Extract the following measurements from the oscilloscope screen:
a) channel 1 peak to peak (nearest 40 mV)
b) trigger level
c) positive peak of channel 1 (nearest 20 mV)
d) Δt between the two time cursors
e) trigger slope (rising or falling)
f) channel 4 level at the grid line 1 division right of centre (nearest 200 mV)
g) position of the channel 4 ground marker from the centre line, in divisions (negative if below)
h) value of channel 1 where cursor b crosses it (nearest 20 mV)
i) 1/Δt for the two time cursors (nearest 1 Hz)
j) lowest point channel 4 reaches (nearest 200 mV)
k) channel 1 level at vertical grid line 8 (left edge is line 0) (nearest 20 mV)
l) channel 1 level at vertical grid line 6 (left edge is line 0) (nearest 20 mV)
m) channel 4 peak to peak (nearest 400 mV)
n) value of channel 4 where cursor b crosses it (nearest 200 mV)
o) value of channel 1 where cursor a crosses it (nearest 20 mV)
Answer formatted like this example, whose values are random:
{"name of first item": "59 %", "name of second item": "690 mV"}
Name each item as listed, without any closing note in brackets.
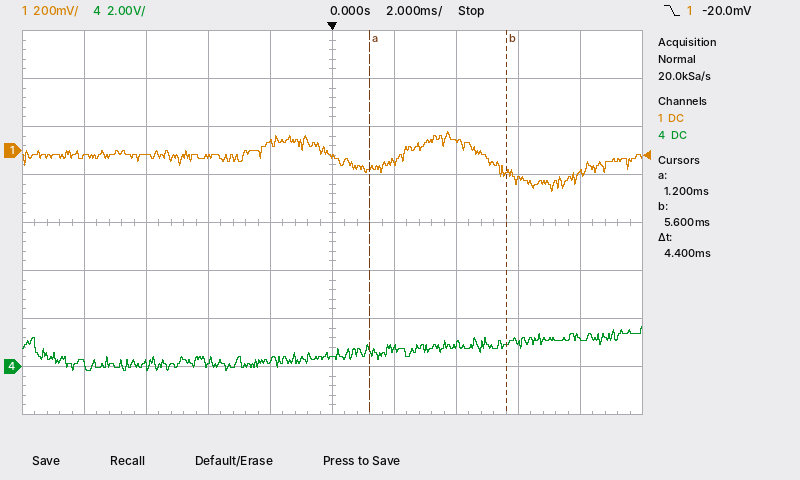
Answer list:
{"channel 1 peak to peak": "240 mV", "trigger level": "-20.0 mV", "positive peak of channel 1": "80 mV", "Δt between the two time cursors": "4.4 ms", "trigger slope": "falling", "channel 4 level at the grid line 1 division right of centre": "800 mV", "position of the channel 4 ground marker from the centre line, in divisions": "-3.0 div", "value of channel 1 where cursor b crosses it": "-100 mV", "1/Δt for the two time cursors": "227 Hz", "lowest point channel 4 reaches": "-200 mV", "channel 1 level at vertical grid line 8 (left edge is line 0)": "-120 mV", "channel 1 level at vertical grid line 6 (left edge is line 0)": "-40 mV", "channel 4 peak to peak": "2.0 V", "value of channel 4 where cursor b crosses it": "1.0 V", "value of channel 1 where cursor a crosses it": "-80 mV"}
